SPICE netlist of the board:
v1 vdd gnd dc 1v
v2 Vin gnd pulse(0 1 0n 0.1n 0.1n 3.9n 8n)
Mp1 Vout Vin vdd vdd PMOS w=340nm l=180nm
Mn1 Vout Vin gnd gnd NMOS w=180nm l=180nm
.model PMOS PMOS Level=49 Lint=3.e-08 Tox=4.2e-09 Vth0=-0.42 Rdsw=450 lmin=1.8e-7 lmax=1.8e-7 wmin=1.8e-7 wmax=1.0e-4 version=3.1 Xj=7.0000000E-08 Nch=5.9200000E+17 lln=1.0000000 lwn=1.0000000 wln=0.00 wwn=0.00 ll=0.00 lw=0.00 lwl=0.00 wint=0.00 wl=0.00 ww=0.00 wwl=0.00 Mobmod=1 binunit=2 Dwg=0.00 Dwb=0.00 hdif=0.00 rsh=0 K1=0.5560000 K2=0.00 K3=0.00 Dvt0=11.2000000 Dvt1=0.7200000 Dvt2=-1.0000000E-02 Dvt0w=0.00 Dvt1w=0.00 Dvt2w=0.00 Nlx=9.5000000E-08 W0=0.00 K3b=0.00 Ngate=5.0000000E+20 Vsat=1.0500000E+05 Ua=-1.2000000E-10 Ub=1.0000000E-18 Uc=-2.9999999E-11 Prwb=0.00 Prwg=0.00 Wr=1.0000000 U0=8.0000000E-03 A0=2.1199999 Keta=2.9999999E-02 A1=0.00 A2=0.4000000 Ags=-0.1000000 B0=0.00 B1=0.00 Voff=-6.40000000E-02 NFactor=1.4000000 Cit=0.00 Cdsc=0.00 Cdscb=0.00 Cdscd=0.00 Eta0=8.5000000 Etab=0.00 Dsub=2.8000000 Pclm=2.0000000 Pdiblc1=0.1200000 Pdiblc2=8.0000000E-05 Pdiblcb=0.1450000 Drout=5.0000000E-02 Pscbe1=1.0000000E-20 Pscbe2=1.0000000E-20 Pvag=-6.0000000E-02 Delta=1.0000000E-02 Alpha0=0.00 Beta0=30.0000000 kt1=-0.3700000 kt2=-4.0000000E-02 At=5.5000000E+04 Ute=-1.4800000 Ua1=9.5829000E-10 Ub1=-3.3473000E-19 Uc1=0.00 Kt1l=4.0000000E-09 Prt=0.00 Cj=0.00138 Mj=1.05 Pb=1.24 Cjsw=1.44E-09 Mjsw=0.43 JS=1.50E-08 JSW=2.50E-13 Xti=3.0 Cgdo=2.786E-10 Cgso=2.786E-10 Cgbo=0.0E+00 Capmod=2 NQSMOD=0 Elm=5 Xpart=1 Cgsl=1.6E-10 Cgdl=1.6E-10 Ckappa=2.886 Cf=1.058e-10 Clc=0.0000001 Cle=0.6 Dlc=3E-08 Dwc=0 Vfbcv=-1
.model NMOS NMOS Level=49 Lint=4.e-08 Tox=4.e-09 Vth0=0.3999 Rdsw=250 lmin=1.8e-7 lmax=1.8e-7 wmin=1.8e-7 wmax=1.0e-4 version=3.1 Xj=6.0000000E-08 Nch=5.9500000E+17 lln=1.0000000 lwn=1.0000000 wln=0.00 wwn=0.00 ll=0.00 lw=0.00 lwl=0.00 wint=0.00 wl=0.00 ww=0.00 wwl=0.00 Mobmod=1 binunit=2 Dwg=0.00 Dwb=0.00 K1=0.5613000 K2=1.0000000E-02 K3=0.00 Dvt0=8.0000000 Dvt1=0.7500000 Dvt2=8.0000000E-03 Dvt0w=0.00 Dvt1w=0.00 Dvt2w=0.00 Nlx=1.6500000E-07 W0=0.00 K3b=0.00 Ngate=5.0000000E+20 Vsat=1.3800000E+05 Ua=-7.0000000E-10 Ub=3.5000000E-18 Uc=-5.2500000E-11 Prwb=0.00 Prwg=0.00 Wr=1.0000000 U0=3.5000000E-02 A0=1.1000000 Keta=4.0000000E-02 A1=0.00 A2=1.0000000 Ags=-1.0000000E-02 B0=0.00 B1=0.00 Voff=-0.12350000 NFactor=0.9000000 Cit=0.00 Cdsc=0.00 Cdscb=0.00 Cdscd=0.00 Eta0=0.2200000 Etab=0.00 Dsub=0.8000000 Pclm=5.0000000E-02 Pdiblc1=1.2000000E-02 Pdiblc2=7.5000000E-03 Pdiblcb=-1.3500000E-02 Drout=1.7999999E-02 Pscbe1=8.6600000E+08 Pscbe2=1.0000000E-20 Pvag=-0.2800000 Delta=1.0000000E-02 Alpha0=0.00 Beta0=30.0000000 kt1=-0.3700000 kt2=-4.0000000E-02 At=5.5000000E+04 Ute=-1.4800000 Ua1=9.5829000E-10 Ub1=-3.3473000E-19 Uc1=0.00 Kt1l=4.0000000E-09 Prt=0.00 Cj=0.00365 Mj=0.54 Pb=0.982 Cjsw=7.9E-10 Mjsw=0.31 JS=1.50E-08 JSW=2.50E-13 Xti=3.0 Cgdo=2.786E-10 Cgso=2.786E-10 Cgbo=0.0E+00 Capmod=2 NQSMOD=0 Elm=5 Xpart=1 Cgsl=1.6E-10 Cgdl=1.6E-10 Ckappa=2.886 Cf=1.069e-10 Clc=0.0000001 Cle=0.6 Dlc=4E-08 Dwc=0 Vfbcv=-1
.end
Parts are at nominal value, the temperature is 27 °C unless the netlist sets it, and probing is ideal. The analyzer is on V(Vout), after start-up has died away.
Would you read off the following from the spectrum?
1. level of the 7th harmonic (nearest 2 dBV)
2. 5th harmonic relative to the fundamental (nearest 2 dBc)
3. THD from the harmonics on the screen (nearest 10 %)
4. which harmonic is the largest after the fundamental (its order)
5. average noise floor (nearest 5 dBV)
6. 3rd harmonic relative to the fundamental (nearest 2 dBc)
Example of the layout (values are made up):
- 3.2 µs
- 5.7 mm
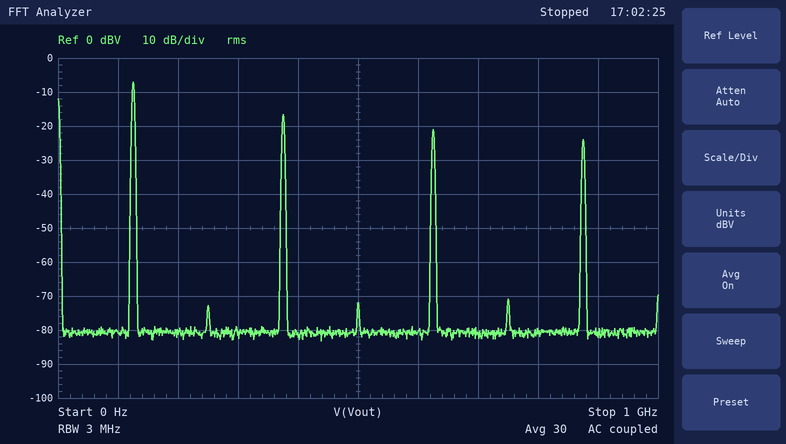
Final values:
- -24 dBV
- -14 dBc
- 40 %
- 3
- -80 dBV
- -10 dBc
